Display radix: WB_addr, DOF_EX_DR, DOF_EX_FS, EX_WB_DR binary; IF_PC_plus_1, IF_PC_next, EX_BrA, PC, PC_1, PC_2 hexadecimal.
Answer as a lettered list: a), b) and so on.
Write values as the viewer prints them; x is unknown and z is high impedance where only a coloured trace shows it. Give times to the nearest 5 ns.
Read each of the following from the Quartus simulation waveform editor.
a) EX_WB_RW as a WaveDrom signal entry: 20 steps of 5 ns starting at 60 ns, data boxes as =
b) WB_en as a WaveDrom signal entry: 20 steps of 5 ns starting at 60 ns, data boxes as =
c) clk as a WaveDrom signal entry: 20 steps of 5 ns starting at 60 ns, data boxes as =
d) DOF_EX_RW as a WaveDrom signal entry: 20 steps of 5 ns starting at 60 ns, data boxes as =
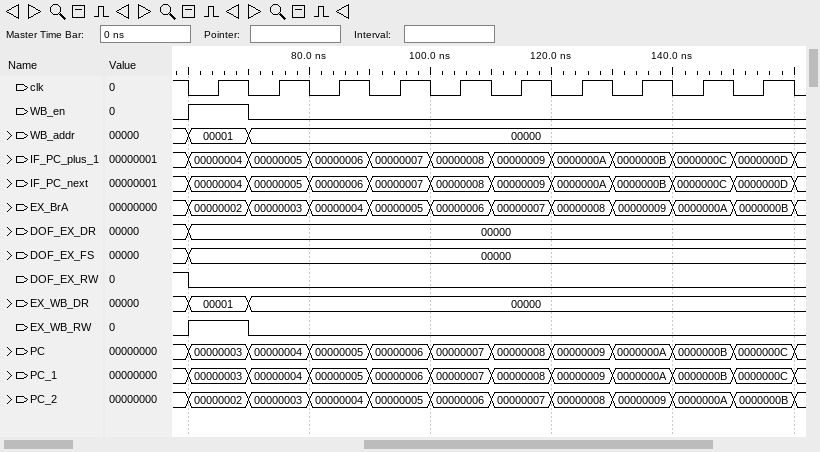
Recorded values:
a) {name: 'EX_WB_RW', wave: '1.0.................'}
b) {name: 'WB_en', wave: '1.0.................'}
c) {name: 'clk', wave: '01010101010101010101'}
d) {name: 'DOF_EX_RW', wave: '0...................'}
